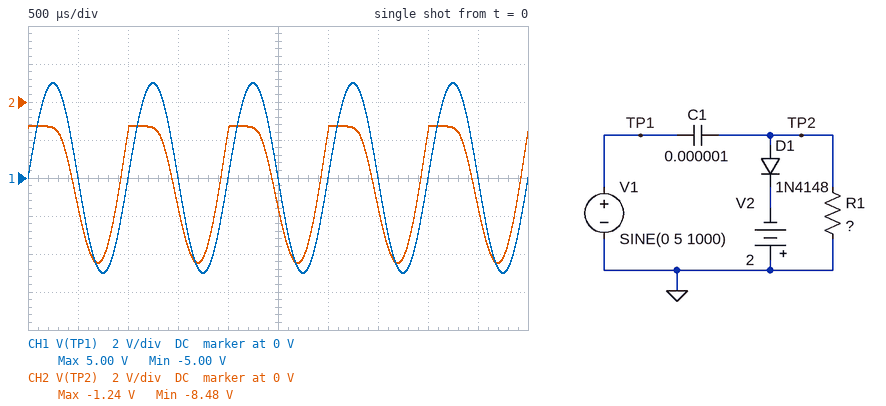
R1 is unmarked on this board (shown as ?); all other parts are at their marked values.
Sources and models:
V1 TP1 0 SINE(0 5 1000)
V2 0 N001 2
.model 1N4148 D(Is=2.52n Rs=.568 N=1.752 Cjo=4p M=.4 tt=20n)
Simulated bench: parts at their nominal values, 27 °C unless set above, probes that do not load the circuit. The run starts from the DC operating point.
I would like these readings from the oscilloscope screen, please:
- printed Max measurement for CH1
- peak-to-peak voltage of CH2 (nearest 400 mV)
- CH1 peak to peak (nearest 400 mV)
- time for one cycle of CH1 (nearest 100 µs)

5.00 V
7.2 V
10.0 V
1.0 ms
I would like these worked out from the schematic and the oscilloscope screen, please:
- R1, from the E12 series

820 Ω
